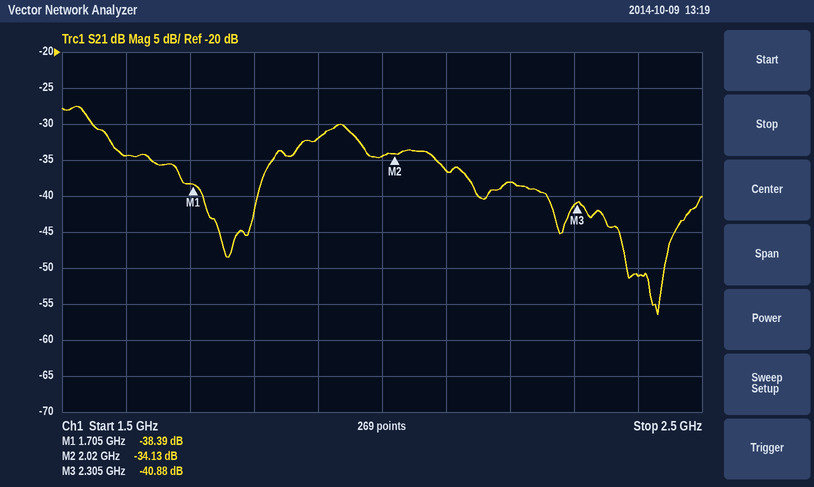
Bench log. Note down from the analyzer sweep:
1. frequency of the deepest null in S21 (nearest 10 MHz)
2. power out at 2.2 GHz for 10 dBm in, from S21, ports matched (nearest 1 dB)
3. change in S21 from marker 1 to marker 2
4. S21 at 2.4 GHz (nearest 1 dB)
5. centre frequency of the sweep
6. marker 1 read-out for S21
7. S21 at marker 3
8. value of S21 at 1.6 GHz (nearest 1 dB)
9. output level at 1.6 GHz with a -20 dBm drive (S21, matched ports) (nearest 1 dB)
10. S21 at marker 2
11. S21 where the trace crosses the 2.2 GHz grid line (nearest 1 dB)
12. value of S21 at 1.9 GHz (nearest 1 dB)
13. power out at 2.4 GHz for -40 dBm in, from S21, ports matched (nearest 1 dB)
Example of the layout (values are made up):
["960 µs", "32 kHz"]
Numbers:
["2.43 GHz", "-28 dBm", "4.26 dB", "-51 dB", "2 GHz", "-38.39 dB", "-40.88 dB", "-34 dB", "-54 dBm", "-34.13 dB", "-38 dB", "-32 dB", "-91 dBm"]
